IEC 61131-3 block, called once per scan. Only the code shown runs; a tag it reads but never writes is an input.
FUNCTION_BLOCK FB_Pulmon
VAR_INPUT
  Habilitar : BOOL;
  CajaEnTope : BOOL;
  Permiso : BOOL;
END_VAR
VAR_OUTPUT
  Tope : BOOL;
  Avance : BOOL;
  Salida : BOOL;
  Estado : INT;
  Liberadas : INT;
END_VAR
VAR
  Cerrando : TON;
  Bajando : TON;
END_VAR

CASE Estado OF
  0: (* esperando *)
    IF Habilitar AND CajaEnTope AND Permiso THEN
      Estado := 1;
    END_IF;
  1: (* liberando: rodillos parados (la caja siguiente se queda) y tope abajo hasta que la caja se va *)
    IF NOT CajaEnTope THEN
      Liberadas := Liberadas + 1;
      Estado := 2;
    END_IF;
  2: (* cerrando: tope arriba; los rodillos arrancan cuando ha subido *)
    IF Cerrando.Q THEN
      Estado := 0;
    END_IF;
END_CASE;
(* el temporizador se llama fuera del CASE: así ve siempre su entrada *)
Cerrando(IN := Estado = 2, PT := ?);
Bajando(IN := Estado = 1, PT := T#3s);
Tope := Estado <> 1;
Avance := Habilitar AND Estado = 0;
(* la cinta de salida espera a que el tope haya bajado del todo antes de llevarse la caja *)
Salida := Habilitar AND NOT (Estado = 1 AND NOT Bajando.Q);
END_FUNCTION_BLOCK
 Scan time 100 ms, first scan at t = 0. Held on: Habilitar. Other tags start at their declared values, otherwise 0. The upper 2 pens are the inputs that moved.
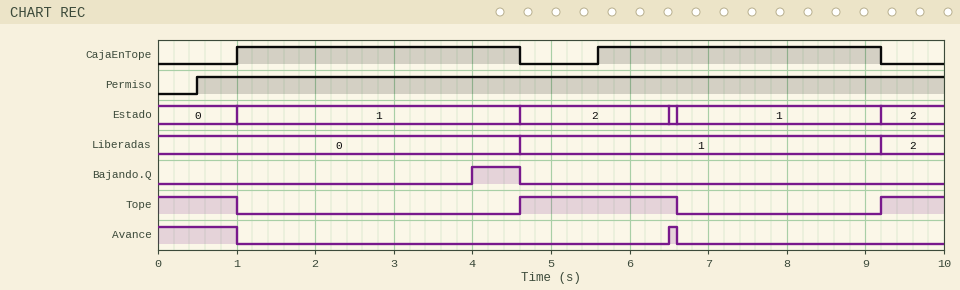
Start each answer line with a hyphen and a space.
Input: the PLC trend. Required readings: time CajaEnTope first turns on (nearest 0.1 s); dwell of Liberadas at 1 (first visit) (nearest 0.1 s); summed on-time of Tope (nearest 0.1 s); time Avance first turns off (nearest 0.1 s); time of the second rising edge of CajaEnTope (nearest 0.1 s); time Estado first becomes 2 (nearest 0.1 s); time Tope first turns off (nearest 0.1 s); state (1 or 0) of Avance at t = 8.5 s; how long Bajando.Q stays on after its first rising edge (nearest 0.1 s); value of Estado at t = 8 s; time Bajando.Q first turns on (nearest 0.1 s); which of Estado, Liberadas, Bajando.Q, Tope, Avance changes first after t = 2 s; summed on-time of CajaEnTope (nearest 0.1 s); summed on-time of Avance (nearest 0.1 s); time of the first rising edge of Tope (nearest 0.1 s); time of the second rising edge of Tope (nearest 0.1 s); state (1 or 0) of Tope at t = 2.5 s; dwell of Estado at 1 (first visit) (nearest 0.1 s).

- 1.0 s
- 4.6 s
- 3.8 s
- 1.0 s
- 5.6 s
- 4.6 s
- 1.0 s
- 0
- 0.6 s
- 1
- 4.0 s
- Bajando.Q
- 7.2 s
- 1.1 s
- 4.6 s
- 9.2 s
- 0
- 3.6 s
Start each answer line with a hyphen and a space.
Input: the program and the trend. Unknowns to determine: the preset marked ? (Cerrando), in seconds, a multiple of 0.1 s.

- 1.8 s
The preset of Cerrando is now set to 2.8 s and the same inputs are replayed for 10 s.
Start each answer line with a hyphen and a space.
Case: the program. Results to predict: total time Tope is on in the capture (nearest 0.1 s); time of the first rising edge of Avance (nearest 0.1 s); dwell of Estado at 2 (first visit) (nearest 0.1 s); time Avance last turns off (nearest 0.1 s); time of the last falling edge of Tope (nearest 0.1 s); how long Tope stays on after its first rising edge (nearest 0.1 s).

- 4.8 s
- 7.5 s
- 2.9 s
- 7.6 s
- 7.6 s
- 3.0 s
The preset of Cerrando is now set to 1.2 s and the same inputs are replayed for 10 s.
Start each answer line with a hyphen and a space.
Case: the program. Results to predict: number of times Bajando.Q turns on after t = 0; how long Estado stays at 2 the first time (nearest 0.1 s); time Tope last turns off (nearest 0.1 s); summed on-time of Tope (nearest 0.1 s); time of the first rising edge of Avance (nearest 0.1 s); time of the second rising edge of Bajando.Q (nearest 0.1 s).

- 2
- 1.3 s
- 6.0 s
- 3.2 s
- 5.9 s
- 9.0 s
